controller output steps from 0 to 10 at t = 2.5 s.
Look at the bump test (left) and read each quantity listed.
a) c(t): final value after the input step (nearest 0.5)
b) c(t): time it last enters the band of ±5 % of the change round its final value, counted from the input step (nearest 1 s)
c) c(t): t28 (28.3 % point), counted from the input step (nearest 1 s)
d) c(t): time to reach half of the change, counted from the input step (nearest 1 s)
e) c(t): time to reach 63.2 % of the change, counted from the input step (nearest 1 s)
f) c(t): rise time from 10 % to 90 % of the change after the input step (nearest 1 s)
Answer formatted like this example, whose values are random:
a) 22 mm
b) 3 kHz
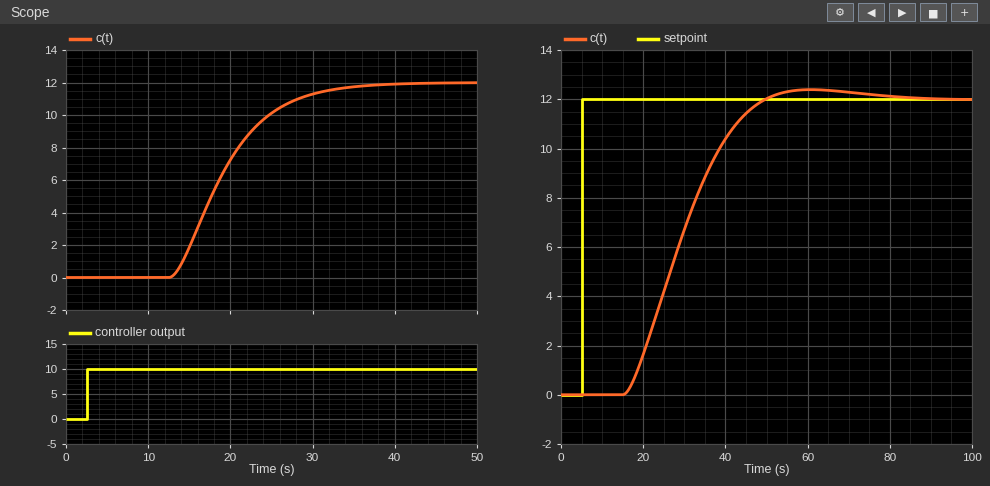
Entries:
a) 12.0
b) 28 s
c) 14 s
d) 16 s
e) 18 s
f) 13 s
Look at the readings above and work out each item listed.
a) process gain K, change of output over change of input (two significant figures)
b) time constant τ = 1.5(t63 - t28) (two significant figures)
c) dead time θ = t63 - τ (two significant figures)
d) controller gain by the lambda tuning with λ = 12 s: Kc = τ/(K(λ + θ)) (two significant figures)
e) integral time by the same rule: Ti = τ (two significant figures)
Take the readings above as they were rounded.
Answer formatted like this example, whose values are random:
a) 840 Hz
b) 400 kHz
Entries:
a) 1.2
b) 6.0 s
c) 12 s
d) 0.21
e) 6.0 s
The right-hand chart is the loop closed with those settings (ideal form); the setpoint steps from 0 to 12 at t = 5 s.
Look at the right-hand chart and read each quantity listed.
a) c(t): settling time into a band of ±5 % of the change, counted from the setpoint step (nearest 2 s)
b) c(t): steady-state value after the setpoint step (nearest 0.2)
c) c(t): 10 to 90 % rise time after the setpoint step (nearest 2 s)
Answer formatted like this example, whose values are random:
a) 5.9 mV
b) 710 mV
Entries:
a) 40 s
b) 12.0
c) 22 s
